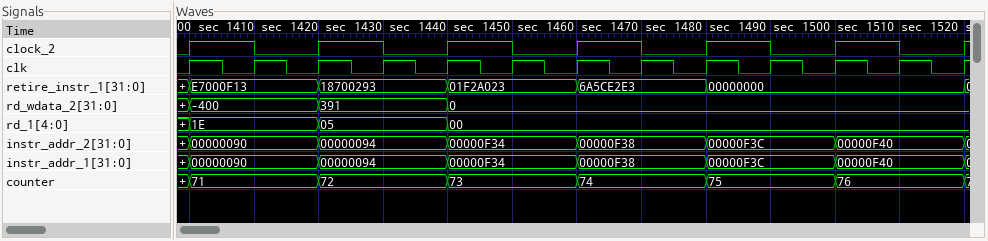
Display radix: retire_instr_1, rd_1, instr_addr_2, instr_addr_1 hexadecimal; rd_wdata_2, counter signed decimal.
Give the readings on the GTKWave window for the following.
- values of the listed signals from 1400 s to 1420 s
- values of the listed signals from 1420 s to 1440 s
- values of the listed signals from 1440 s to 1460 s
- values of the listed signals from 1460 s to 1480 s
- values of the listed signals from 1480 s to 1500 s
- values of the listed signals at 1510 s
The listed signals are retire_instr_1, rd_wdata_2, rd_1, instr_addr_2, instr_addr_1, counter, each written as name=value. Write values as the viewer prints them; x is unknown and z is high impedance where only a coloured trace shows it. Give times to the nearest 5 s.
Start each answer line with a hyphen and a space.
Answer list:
- retire_instr_1=E7000F13, rd_wdata_2=-400, rd_1=1E, instr_addr_2=00000090, instr_addr_1=00000090, counter=71
- retire_instr_1=18700293, rd_wdata_2=391, rd_1=05, instr_addr_2=00000094, instr_addr_1=00000094, counter=72
- retire_instr_1=01F2A023, rd_wdata_2=0, rd_1=00, instr_addr_2=00000F34, instr_addr_1=00000F34, counter=73
- retire_instr_1=6A5CE2E3, rd_wdata_2=0, rd_1=00, instr_addr_2=00000F38, instr_addr_1=00000F38, counter=74
- retire_instr_1=00000000, rd_wdata_2=0, rd_1=00, instr_addr_2=00000F3C, instr_addr_1=00000F3C, counter=75
- retire_instr_1=00000000, rd_wdata_2=0, rd_1=00, instr_addr_2=00000F40, instr_addr_1=00000F40, counter=76
